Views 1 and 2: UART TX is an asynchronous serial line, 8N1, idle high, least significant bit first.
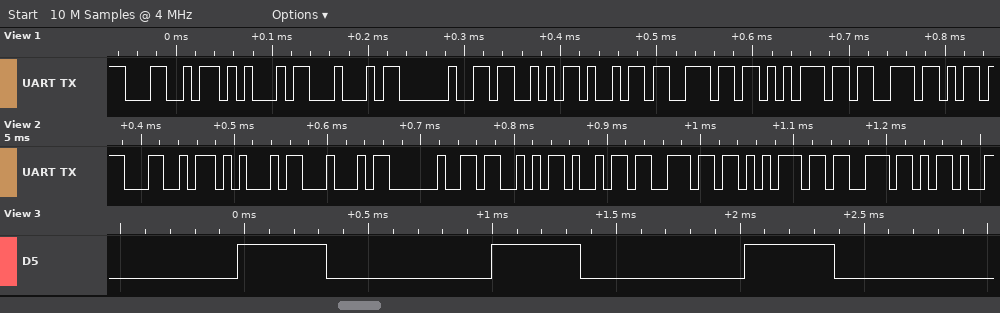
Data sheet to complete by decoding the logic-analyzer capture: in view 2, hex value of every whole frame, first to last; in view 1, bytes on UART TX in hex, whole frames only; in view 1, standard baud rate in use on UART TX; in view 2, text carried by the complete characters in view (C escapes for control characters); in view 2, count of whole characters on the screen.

4C 45 44 20 53 69 6E 75 73 2D
4C 45 44 20 53 69 6E 75 73
115200 baud
"LED Sinus-"
10
